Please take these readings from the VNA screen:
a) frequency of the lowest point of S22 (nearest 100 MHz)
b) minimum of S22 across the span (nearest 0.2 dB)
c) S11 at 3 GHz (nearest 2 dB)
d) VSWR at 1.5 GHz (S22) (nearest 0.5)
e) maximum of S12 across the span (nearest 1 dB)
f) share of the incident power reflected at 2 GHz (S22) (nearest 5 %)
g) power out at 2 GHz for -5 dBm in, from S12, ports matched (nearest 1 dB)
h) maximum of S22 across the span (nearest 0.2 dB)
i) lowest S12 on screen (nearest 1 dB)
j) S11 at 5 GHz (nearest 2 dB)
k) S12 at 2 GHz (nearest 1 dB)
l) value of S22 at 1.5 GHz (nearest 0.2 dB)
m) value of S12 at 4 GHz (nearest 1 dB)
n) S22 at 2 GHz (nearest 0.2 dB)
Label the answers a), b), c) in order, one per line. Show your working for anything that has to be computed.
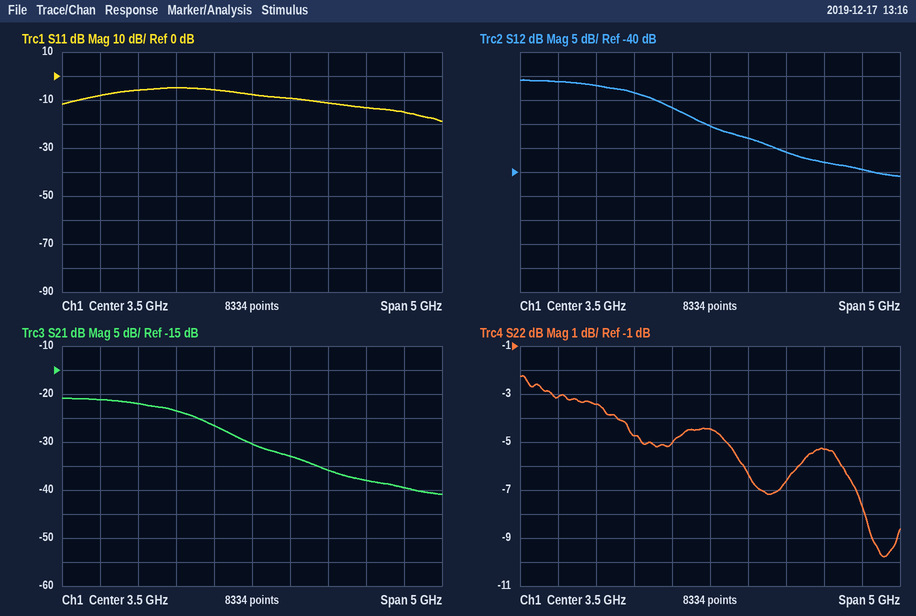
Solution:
a) 5.8 GHz
b) -9.8 dB
c) -6 dB
d) |Γ| = 10^(-3.2/20) = 0.6918; VSWR = (1 + 0.6918)/(1 − 0.6918) ≈ 5.5
e) -21 dB
f) 10^(-3.4/10) ≈ 45.7 %, so 45 % to the nearest 5 %
g) -5 dBm + (-22 dB) = -27 dBm
h) -2.2 dB
i) -41 dB
j) -14 dB
k) -22 dB
l) -3.2 dB
m) -33 dB
n) -3.4 dB
